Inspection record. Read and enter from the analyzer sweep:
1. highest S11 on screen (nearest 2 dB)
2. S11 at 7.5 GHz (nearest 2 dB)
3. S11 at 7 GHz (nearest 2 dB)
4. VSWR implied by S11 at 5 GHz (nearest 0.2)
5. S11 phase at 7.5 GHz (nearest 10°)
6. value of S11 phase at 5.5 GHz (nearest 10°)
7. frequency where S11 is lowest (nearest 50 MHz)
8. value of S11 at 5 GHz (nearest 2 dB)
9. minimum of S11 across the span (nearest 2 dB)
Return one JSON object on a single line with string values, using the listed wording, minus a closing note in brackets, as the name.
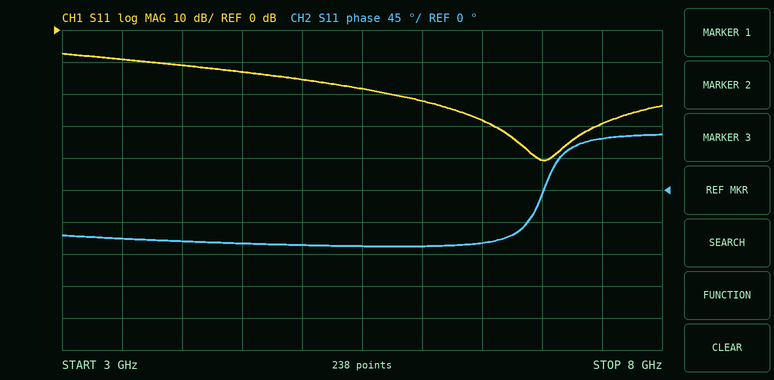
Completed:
{"highest S11 on screen": "-8 dB", "S11 at 7.5 GHz": "-30 dB", "S11 at 7 GHz": "-40 dB", "VSWR implied by S11 at 5 GHz": "1.4", "S11 phase at 7.5 GHz": "70°", "value of S11 phase at 5.5 GHz": "-80°", "frequency where S11 is lowest": "7.00 GHz", "value of S11 at 5 GHz": "-16 dB", "minimum of S11 across the span": "-40 dB"}
